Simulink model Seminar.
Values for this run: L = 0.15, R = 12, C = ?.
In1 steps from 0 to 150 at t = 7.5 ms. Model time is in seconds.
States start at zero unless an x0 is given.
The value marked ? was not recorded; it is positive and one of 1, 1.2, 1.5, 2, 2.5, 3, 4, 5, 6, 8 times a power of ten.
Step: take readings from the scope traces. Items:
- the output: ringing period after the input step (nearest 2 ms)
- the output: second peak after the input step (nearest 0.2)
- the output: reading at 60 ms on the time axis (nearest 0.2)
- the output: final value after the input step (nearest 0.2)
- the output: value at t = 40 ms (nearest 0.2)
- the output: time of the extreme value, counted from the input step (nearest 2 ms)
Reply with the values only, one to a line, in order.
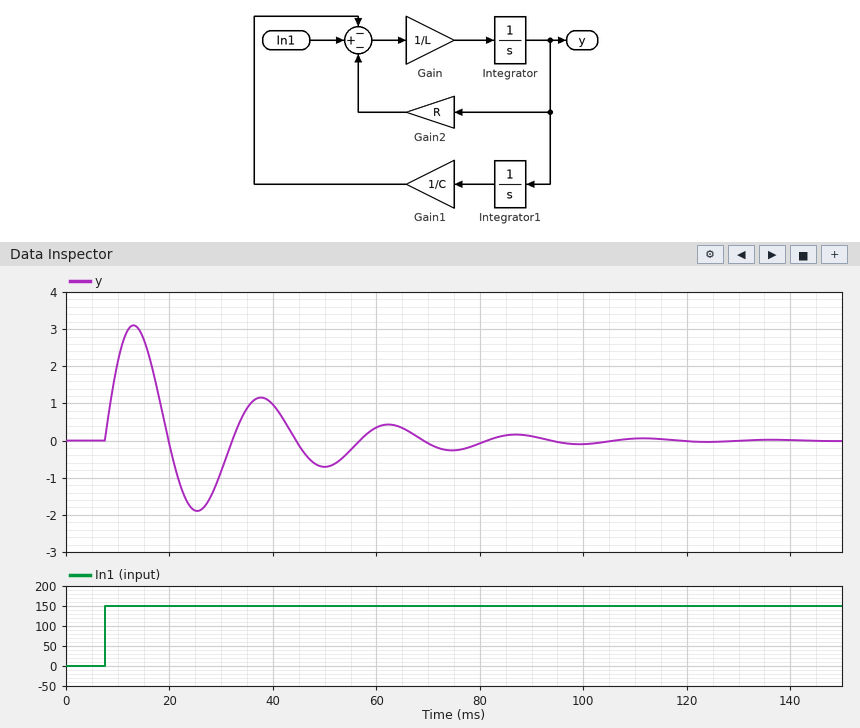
24 ms
1.2
0.4
0.0
1.0
6 ms
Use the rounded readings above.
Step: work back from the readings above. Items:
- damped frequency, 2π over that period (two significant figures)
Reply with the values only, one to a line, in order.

0.26 rad/ms
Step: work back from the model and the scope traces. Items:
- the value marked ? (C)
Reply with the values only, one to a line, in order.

0.0001
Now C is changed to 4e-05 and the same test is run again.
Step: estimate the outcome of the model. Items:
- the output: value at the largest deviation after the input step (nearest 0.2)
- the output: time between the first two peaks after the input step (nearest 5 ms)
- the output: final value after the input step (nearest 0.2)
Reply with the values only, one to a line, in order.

2.2
15 ms
0.0
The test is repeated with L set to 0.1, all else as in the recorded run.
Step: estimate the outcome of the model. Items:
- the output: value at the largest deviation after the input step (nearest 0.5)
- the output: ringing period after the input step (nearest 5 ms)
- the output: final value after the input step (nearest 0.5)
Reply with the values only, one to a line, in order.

3.5
20 ms
0.0
